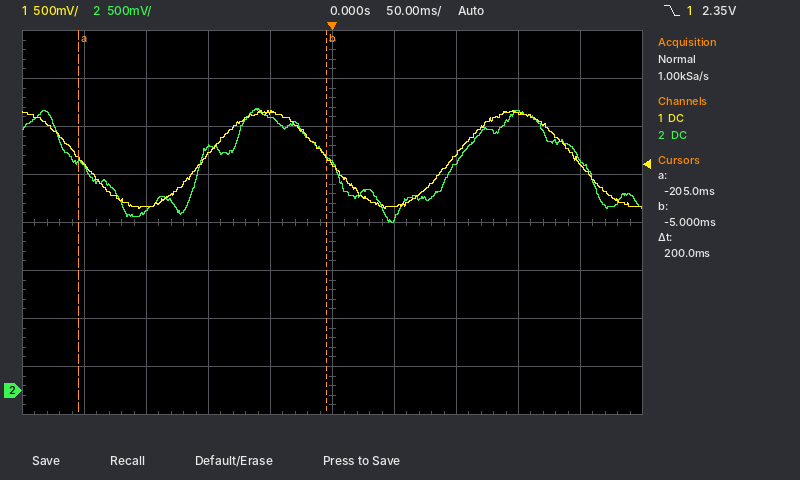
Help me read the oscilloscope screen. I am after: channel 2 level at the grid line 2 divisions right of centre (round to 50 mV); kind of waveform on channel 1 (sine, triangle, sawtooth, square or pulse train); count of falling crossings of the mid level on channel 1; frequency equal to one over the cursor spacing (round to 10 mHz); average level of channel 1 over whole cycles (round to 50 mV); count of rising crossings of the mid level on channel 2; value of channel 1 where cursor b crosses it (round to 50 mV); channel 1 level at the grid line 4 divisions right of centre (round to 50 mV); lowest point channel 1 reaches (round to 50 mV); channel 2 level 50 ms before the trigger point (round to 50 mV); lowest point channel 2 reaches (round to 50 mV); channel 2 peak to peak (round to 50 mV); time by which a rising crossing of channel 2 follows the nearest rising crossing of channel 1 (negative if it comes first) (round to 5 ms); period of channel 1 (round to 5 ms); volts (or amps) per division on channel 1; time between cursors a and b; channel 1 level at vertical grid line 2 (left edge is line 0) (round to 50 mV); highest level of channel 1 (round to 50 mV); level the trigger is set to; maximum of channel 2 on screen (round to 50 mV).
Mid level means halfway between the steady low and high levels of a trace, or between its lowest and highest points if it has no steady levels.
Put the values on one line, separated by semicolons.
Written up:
2.40 V; sine; 3; 5.00 Hz; 2.40 V; 2; 2.45 V; 2.35 V; 1.90 V; 2.85 V; 1.75 V; 1.20 V; 0 ms; 200 ms; 500 mV; 200 ms; 1.90 V; 2.90 V; 2.35 V; 2.95 V
